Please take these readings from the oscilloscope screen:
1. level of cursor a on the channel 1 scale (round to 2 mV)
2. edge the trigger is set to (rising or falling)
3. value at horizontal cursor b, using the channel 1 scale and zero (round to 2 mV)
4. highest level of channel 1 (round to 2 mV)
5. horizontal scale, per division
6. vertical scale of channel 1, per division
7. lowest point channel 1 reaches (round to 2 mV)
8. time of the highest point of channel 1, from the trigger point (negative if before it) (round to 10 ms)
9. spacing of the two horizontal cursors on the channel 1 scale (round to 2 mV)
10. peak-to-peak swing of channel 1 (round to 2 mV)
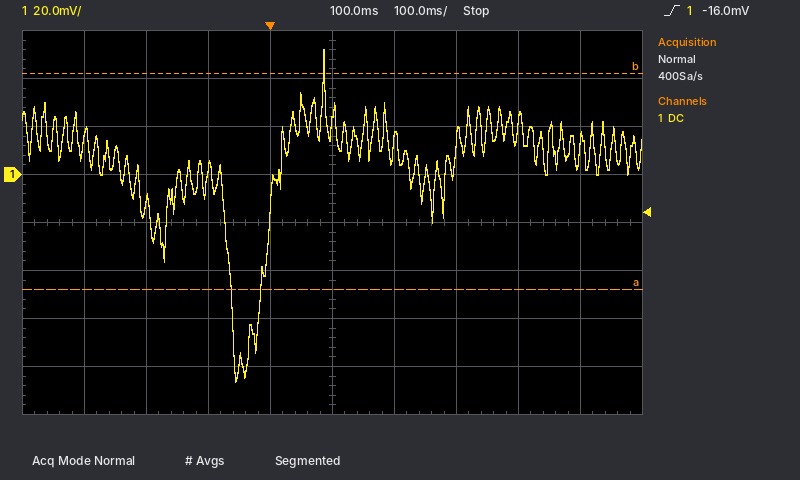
-48 mV
rising
42 mV
52 mV
100 ms
20 mV
-86 mV
+90 ms
90 mV
138 mV
